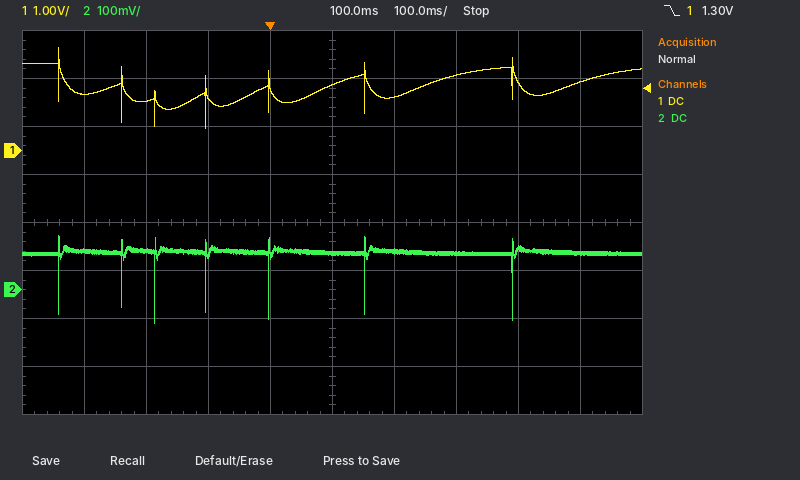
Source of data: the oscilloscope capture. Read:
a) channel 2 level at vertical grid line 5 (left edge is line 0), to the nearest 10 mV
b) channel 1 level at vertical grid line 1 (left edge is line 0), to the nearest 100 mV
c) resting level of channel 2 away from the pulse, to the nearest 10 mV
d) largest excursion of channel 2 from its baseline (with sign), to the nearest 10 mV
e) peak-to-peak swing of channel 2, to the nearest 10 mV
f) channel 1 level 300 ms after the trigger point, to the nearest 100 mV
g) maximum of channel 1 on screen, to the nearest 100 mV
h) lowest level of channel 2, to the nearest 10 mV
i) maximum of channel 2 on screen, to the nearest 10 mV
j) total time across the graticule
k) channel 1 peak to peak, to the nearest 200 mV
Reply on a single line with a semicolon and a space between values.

80 mV; 1.2 V; 80 mV; -150 mV; 180 mV; 1.6 V; 2.1 V; -70 mV; 110 mV; 1 s; 1.6 V
